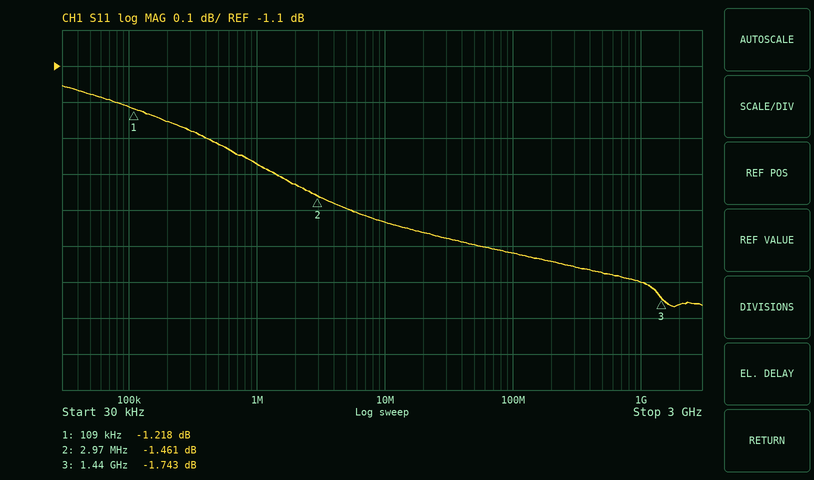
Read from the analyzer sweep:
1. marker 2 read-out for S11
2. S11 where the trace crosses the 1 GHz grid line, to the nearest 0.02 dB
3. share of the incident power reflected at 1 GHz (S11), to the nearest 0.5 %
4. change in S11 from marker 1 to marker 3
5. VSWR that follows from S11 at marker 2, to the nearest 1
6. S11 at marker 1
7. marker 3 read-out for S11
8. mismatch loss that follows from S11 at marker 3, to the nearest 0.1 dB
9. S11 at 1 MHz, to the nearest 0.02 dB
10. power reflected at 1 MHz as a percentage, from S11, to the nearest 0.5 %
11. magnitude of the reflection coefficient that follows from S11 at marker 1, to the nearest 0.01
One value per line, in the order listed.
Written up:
-1.461 dB
-1.70 dB
67.5 %
-0.525 dB
12
-1.218 dB
-1.743 dB
4.8 dB
-1.38 dB
73.0 %
0.87
